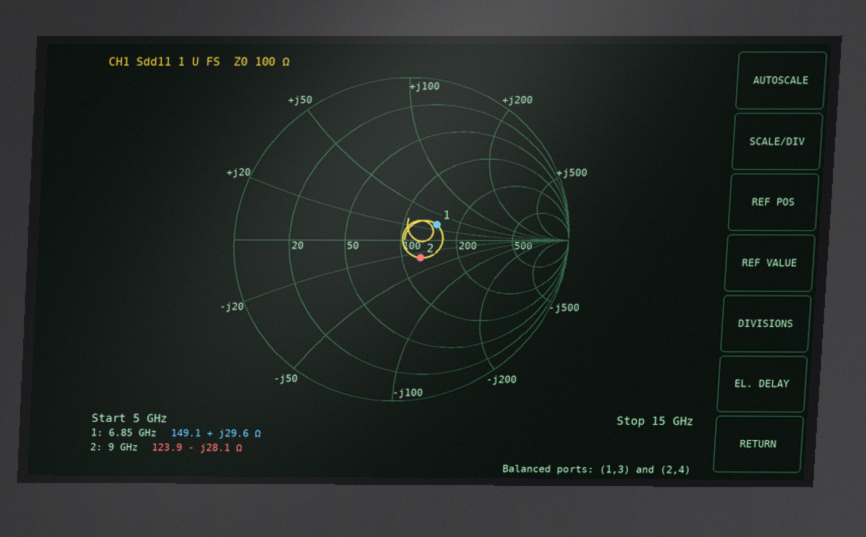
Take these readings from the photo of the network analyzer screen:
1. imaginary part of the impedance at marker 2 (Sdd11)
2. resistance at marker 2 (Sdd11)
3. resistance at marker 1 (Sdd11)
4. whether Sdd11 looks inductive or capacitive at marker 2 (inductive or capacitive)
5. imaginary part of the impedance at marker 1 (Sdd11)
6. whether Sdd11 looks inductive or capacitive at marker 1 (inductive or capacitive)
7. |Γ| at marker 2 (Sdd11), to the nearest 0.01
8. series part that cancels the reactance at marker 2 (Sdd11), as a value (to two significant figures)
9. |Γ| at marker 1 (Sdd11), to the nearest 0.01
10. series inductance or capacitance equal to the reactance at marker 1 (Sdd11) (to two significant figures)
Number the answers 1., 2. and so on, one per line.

1. -28.1 Ω
2. 123.9 Ω
3. 149.1 Ω
4. capacitive
5. +29.6 Ω
6. inductive
7. 0.16
8. 500 pH
9. 0.23
10. 690 pH
